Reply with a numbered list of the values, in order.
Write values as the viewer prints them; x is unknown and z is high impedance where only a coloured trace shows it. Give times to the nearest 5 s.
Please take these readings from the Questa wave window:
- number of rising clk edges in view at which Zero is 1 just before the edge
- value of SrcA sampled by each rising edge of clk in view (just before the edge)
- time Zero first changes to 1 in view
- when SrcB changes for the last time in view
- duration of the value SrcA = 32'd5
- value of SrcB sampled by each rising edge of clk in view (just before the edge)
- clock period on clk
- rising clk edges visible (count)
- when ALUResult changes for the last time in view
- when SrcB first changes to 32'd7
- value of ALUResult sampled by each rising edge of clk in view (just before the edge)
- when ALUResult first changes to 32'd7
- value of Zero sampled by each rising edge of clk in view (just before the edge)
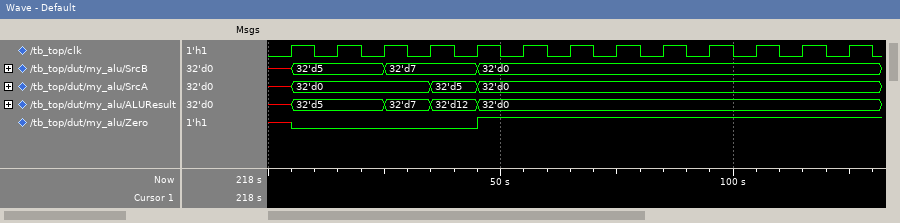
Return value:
1. 8
2. x, 32'd0, 32'd0, 32'd0, 32'd5, 32'd0, 32'd0, 32'd0, 32'd0, 32'd0, 32'd0, 32'd0, 32'd0
3. 45 s
4. 45 s
5. 10 s
6. x, 32'd5, 32'd5, 32'd7, 32'd7, 32'd0, 32'd0, 32'd0, 32'd0, 32'd0, 32'd0, 32'd0, 32'd0
7. 10 s
8. 13
9. 45 s
10. 25 s
11. x, 32'd5, 32'd5, 32'd7, 32'd12, 32'd0, 32'd0, 32'd0, 32'd0, 32'd0, 32'd0, 32'd0, 32'd0
12. 25 s
13. x 0 0 0 0 1 1 1 1 1 1 1 1
